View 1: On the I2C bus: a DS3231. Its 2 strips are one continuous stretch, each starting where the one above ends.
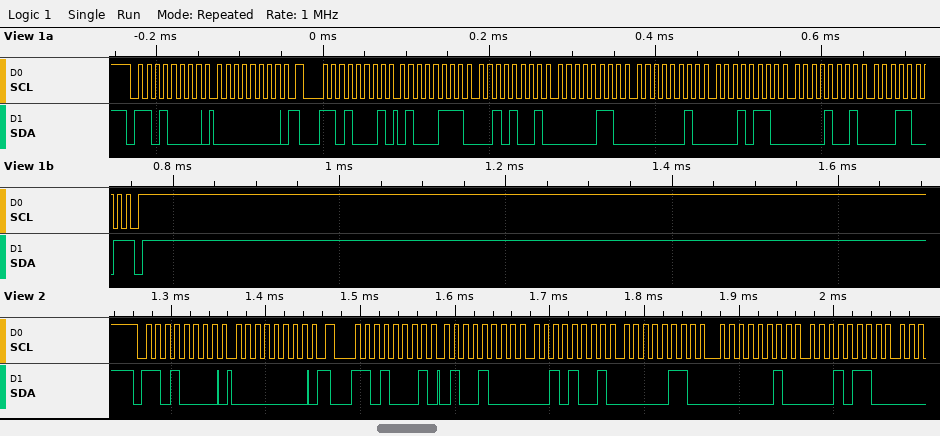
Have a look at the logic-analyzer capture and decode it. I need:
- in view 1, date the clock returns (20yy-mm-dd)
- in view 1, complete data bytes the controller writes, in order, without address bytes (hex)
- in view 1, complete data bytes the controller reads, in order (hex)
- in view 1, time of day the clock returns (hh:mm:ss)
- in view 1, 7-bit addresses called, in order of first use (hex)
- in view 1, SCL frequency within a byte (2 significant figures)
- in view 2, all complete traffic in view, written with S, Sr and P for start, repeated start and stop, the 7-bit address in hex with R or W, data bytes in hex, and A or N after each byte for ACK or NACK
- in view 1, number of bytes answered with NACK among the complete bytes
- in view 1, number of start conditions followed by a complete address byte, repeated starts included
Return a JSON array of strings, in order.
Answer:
["2019-09-16", "00", "47 29 06 02 16 09 19", "06:29:47", "0x68", "100 kHz", "S 68W A 00 A Sr 68R A 48 A 29 A 06 A 02 A 16 A", "1", "2"]
